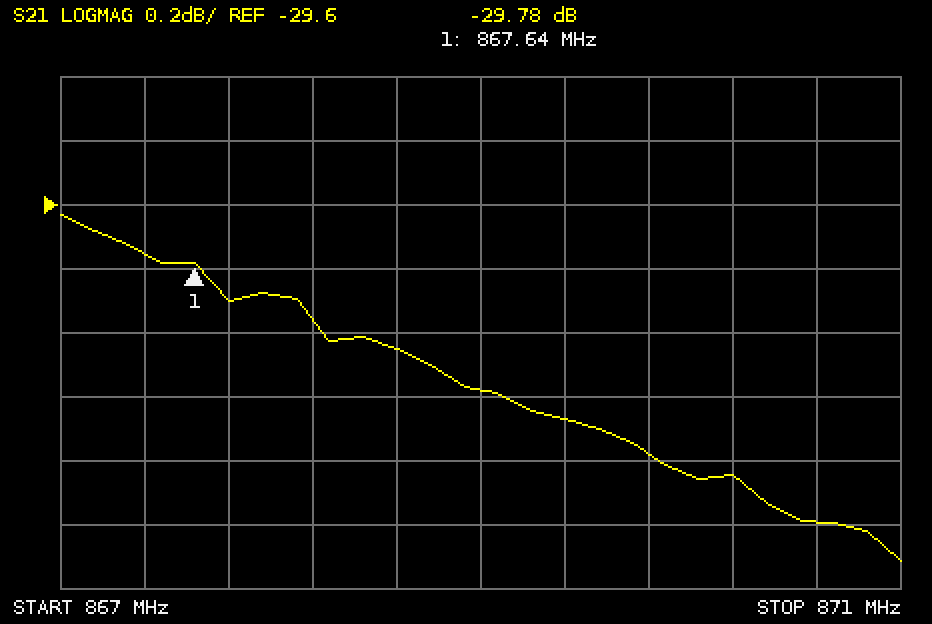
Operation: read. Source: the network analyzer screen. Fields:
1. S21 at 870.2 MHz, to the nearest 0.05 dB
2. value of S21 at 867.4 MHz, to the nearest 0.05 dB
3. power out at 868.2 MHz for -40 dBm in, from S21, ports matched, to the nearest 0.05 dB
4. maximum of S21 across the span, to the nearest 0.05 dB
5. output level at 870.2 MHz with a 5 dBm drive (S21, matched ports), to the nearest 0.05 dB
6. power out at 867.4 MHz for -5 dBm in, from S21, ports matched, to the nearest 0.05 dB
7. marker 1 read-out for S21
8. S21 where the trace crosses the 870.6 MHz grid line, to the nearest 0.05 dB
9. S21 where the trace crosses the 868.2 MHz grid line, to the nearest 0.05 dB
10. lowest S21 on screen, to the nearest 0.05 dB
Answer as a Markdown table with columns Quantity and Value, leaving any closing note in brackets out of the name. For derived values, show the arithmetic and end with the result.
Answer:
| Quantity | Value |
|---|---|
| S21 at 870.2 MHz, to the nearest 0.05 dB | -30.45 dB |
| value of S21 at 867.4 MHz, to the nearest 0.05 dB | -29.75 dB |
| power out at 868.2 MHz for -40 dBm in, from S21, ports matched, to the nearest 0.05 dB | -40 dBm + (-29.95 dB) = -69.95 dBm |
| maximum of S21 across the span, to the nearest 0.05 dB | -29.65 dB |
| output level at 870.2 MHz with a 5 dBm drive (S21, matched ports), to the nearest 0.05 dB | 5 dBm + (-30.45 dB) = -25.45 dBm |
| power out at 867.4 MHz for -5 dBm in, from S21, ports matched, to the nearest 0.05 dB | -5 dBm + (-29.75 dB) = -34.75 dBm |
| marker 1 read-out for S21 | -29.78 dB |
| S21 where the trace crosses the 870.6 MHz grid line, to the nearest 0.05 dB | -30.60 dB |
| S21 where the trace crosses the 868.2 MHz grid line, to the nearest 0.05 dB | -29.95 dB |
| lowest S21 on screen, to the nearest 0.05 dB | -30.70 dB |
